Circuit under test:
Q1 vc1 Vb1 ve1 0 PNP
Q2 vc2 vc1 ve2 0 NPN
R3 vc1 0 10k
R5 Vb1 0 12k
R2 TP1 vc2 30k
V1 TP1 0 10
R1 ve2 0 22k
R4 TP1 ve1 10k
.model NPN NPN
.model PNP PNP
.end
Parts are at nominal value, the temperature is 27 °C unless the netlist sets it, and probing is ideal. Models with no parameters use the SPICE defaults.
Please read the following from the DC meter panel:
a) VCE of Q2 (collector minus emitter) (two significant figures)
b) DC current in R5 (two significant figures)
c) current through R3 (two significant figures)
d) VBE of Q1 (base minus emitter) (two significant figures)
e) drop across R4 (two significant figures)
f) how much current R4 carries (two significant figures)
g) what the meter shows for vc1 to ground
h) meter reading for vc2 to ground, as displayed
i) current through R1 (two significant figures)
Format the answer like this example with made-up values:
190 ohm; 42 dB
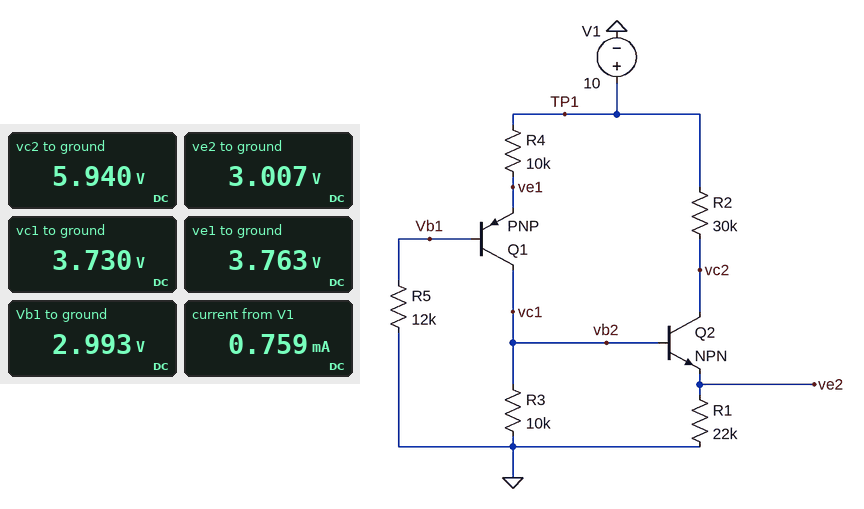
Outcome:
2.9 V; 250 µA; 370 µA; -770 mV; 6.2 V; 620 µA; 3.730 V; 5.940 V; 140 µA
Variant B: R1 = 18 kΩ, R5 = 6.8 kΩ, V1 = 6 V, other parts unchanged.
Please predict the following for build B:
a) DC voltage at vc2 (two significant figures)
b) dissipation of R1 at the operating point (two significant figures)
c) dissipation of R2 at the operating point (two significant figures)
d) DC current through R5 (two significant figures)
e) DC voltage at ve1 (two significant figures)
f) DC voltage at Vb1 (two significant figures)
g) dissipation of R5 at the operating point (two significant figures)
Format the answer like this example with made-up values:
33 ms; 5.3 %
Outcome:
3.8 V; 97 µW; 160 µW; 190 µA; 2.1 V; 1.3 V; 250 µW
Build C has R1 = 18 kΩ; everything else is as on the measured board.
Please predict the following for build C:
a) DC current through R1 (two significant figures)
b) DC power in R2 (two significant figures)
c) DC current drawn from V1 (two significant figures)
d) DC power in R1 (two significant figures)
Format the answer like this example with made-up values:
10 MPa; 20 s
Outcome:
170 µA; 820 µW; 790 µA; 500 µW
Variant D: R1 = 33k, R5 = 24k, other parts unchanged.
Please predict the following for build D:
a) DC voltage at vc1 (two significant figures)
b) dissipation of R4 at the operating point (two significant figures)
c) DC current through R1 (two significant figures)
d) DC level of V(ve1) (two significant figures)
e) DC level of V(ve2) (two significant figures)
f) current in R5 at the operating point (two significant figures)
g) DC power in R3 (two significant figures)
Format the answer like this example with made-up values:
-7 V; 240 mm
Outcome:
4.2 V; 3.3 mW; 110 µA; 4.3 V; 3.5 V; 150 µA; 1.8 mW
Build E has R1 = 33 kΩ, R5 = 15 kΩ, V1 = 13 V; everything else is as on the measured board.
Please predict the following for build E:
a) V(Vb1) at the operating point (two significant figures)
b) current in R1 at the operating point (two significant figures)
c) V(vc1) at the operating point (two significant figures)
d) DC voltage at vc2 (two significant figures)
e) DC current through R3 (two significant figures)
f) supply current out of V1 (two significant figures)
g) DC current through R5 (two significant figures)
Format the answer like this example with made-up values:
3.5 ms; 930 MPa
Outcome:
4.3 V; 130 µA; 5.0 V; 9.1 V; 500 µA; 920 µA; 290 µA
